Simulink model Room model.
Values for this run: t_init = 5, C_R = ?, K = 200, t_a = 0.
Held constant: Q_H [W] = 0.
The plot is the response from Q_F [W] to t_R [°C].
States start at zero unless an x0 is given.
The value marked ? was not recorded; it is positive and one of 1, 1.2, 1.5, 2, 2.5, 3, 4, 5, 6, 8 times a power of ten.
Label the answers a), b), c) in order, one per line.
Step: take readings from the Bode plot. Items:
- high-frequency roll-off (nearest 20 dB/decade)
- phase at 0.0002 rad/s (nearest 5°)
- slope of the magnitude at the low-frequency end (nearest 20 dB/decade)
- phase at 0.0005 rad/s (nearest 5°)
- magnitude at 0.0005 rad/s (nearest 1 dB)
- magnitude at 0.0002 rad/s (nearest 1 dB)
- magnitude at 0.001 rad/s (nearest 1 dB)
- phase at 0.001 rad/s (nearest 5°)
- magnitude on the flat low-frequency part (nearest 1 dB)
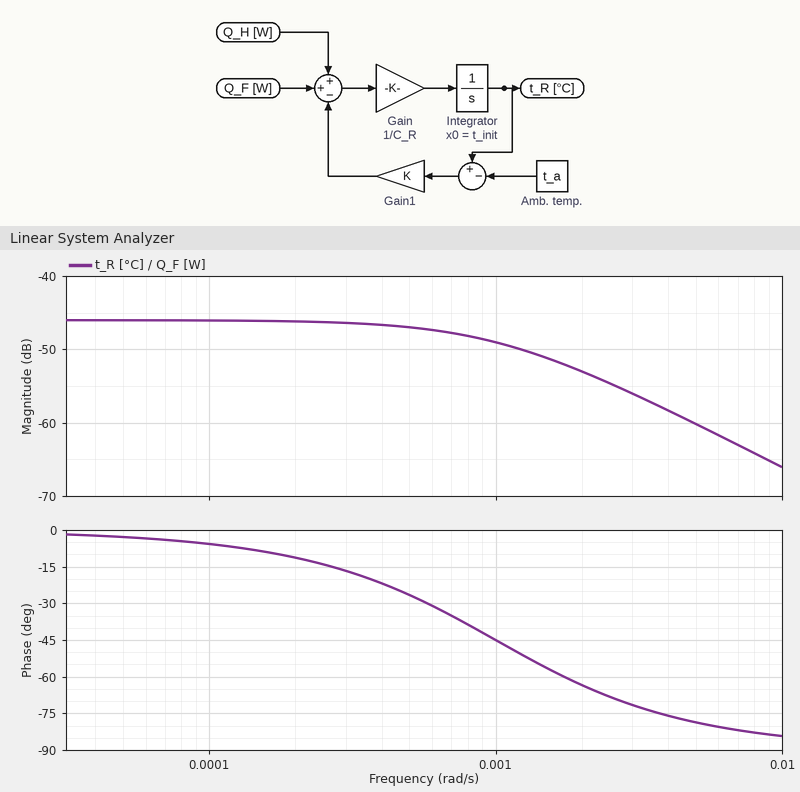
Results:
a) -20 dB/decade
b) -10°
c) 0 dB/decade
d) -25°
e) -47 dB
f) -46 dB
g) -49 dB
h) -45°
i) -46 dB
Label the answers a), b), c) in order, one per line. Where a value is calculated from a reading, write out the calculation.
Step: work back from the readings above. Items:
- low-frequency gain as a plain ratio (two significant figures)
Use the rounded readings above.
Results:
a) 10^(-46 / 20) = 0.0050
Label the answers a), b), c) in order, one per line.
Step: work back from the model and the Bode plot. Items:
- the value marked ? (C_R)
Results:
a) 200000
